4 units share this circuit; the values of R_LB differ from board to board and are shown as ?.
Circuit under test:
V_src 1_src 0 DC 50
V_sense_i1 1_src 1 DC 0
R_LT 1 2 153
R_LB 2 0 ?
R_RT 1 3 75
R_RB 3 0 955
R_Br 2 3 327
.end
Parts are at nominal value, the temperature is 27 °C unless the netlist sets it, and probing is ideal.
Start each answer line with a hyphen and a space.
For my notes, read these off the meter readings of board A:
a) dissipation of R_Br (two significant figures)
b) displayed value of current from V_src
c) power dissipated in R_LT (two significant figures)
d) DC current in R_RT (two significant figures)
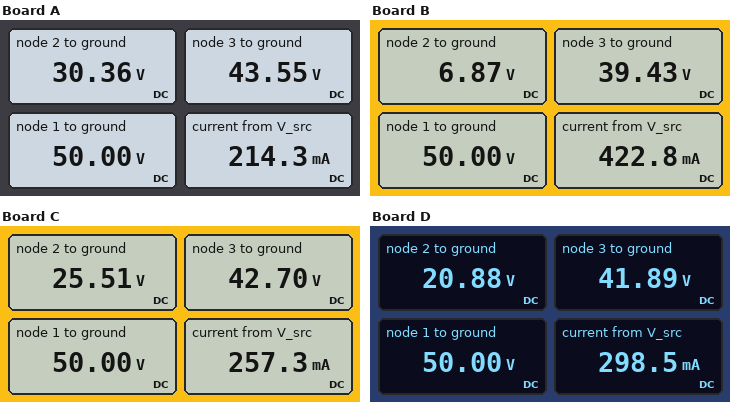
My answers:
- 530 mW
- 214.3 mA
- 2.5 W
- 86 mA
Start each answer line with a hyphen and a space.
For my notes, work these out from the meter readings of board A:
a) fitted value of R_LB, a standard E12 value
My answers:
- 180 Ω
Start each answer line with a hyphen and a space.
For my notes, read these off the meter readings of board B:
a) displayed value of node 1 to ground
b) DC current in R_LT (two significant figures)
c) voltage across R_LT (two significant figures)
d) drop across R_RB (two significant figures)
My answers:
- 50.00 V
- 280 mA
- 43 V
- 39 V
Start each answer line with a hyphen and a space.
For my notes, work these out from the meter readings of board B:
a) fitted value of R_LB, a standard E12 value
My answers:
- 18 Ω
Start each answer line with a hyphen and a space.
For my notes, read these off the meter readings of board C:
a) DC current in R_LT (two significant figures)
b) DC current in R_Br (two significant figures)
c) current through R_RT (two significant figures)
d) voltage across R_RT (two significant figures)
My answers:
- 160 mA
- 53 mA
- 97 mA
- 7.3 V
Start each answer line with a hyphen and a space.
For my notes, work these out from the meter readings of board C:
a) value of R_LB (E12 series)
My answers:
- 120 Ω
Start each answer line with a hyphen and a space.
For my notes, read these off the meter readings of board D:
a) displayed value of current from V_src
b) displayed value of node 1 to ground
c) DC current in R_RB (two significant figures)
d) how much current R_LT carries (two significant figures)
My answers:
- 298.5 mA
- 50.00 V
- 44 mA
- 190 mA
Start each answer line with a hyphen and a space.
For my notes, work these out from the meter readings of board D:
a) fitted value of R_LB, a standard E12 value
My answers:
- 82 Ω
